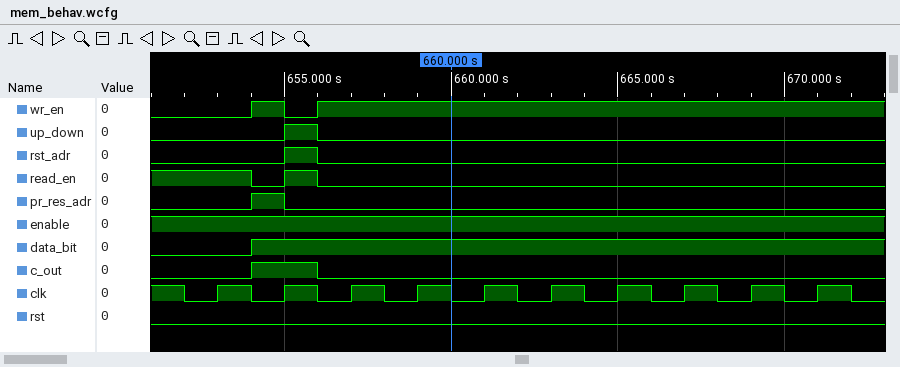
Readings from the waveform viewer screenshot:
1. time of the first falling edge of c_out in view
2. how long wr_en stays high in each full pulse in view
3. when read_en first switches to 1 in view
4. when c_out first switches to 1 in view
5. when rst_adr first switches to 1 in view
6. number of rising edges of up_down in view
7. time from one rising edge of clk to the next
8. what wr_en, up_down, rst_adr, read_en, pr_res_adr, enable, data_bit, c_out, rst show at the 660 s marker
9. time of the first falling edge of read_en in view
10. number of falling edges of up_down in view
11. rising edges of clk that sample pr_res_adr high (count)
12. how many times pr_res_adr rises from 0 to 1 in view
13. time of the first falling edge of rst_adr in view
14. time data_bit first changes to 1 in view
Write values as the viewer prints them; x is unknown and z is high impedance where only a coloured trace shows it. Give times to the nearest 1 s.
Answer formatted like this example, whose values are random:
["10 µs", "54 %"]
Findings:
["656 s", "1 s", "655 s", "654 s", "655 s", "1", "2 s", "wr_en=1, up_down=0, rst_adr=0, read_en=0, pr_res_adr=0, enable=1, data_bit=1, c_out=0, rst=0", "654 s", "1", "1", "1", "656 s", "654 s"]
